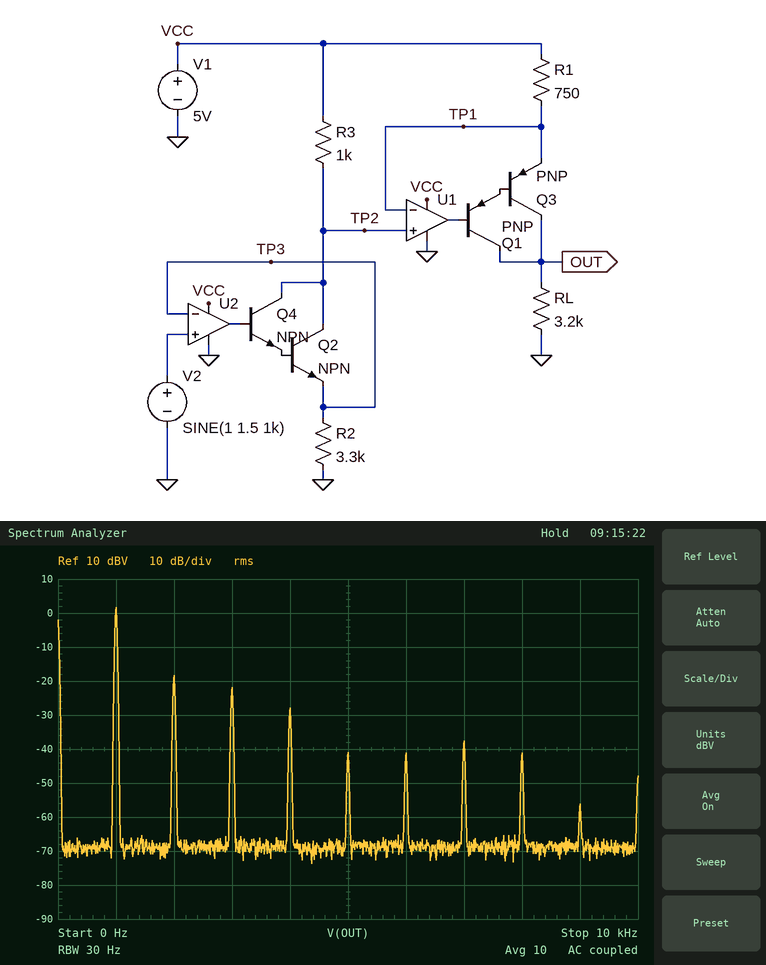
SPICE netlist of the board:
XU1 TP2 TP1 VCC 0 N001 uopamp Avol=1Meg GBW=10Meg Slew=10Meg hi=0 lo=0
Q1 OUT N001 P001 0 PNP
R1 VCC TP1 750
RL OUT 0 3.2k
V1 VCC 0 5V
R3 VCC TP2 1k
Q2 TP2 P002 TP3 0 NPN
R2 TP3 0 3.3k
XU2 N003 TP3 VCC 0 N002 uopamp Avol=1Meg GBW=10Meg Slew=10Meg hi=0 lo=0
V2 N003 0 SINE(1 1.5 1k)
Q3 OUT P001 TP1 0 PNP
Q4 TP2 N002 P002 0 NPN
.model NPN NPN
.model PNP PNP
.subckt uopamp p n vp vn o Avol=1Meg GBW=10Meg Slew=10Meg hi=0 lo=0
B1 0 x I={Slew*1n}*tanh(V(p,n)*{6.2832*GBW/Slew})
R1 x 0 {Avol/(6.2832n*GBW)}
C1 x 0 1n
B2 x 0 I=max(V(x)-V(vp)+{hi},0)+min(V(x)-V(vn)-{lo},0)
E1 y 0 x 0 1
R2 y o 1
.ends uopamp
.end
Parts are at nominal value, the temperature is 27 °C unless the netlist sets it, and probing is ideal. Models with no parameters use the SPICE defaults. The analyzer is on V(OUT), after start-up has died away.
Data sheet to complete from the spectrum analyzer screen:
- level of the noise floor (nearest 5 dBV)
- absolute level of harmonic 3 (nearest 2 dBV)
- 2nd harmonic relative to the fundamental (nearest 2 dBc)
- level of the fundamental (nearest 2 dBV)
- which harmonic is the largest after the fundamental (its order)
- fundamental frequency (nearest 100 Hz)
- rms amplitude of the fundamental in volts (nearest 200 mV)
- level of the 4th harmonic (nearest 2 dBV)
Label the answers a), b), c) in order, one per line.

a) -70 dBV
b) -22 dBV
c) -20 dBc
d) 2 dBV
e) 2
f) 1.0 kHz
g) 1.2 V
h) -28 dBV
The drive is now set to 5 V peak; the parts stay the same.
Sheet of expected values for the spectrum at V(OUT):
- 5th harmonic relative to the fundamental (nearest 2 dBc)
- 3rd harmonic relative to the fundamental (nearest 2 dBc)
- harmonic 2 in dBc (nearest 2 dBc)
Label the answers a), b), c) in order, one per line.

a) -16 dBc
b) -10 dBc
c) -30 dBc
